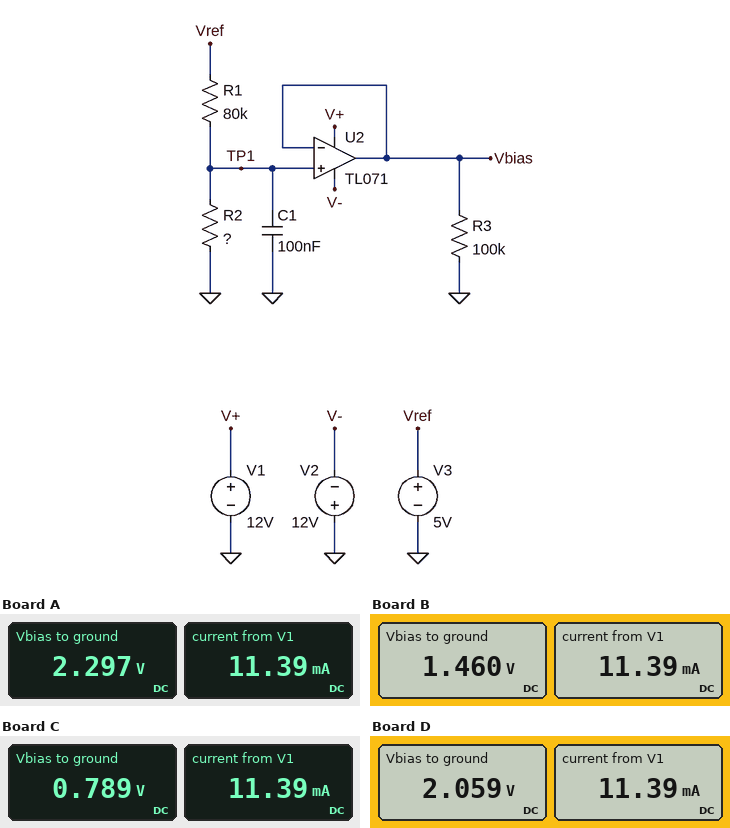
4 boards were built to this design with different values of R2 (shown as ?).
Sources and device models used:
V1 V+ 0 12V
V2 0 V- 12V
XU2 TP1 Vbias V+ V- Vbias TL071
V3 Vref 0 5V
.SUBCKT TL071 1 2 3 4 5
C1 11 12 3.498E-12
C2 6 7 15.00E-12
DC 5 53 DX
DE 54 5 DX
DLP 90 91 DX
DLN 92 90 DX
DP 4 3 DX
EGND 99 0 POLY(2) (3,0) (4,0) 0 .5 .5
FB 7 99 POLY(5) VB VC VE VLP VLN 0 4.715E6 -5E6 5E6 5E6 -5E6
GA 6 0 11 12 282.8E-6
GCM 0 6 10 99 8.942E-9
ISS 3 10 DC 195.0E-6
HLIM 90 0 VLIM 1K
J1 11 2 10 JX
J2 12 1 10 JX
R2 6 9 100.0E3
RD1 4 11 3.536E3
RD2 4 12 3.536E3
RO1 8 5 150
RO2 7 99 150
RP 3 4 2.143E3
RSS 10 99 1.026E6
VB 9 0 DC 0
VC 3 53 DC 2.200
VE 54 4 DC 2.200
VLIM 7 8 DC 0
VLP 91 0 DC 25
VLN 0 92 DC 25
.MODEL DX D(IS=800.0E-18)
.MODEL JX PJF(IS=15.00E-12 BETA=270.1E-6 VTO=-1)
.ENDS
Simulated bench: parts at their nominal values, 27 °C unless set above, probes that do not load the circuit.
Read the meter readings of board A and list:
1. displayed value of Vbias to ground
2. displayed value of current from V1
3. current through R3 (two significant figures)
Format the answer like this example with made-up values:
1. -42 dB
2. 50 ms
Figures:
1. 2.297 V
2. 11.39 mA
3. 23 µA
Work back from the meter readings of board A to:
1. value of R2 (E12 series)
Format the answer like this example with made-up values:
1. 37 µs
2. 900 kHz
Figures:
1. 68 kΩ
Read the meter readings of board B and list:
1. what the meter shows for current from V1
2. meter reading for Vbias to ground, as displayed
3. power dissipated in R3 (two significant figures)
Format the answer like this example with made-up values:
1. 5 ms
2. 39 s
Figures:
1. 11.39 mA
2. 1.460 V
3. 21 µW
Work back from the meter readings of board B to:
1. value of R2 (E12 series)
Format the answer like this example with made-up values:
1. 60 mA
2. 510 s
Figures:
1. 33 kΩ
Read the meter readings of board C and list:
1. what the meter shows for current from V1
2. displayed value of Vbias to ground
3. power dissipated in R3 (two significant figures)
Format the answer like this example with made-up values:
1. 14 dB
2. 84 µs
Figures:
1. 11.39 mA
2. 0.789 V
3. 6.2 µW
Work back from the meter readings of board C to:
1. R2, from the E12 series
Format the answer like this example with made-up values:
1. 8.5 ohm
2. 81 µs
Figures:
1. 15 kΩ
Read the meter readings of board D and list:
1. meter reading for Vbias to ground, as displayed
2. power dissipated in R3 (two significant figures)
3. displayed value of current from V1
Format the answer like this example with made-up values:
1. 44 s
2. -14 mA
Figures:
1. 2.059 V
2. 42 µW
3. 11.39 mA
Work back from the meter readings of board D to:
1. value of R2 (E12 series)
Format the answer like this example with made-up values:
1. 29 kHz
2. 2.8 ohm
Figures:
1. 56 kΩ
